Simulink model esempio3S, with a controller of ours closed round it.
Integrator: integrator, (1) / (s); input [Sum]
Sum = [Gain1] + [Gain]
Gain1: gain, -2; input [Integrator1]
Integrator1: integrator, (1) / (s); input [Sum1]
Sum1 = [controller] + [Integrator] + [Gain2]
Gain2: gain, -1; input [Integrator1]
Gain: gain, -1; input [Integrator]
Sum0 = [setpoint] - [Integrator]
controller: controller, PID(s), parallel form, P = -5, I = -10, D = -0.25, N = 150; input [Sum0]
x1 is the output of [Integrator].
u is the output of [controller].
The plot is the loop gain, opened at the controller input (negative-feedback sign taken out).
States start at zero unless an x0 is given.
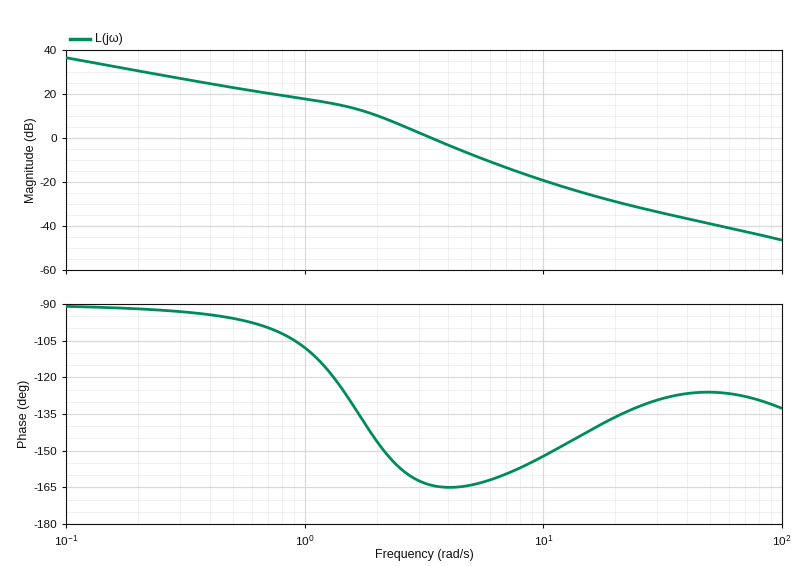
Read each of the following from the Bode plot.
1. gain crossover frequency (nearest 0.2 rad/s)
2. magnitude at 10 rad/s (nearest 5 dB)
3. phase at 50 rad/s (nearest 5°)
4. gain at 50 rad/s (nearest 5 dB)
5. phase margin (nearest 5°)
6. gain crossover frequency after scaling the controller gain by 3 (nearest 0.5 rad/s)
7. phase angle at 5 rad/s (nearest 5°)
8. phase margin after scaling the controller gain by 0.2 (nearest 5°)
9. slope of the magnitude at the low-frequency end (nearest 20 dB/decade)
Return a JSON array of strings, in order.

["3.4 rad/s", "-20 dB", "-125°", "-40 dB", "15°", "5.5 rad/s", "-165°", "50°", "-20 dB/decade"]
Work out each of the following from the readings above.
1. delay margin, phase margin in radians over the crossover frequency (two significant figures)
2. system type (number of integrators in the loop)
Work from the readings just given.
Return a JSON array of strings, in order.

["0.077 s", "1"]
